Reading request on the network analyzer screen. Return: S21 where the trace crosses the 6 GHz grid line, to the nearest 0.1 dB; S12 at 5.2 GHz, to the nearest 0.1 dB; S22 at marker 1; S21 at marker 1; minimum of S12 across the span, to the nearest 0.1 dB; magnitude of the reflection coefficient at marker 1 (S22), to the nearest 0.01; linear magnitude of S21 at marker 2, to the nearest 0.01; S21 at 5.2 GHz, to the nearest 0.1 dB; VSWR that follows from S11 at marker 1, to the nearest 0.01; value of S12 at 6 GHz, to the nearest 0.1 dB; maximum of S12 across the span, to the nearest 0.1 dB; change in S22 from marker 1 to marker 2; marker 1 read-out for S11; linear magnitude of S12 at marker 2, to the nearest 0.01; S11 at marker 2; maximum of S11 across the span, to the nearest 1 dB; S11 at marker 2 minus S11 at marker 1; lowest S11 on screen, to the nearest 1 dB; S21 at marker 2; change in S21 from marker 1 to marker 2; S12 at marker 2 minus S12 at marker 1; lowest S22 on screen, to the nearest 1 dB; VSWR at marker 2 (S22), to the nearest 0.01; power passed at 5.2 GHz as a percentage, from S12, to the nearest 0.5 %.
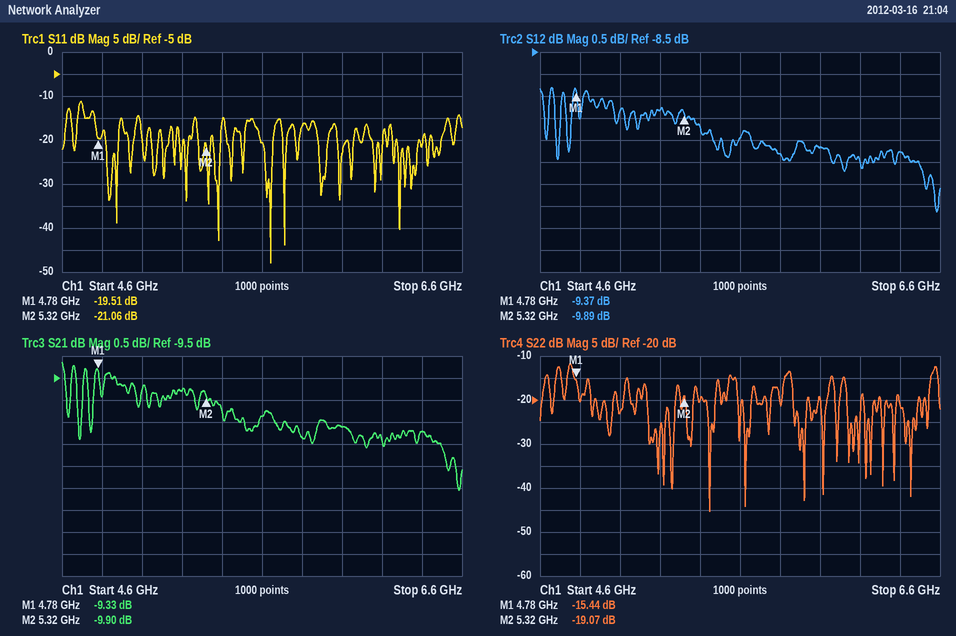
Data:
-10.6 dB
-9.8 dB
-15.44 dB
-9.33 dB
-12.1 dB
0.17
0.32
-9.8 dB
1.24
-10.7 dB
-9.3 dB
-3.63 dB
-19.51 dB
0.32
-21.06 dB
-11 dB
-1.55 dB
-48 dB
-9.90 dB
-0.57 dB
-0.52 dB
-45 dB
1.25
10.5 %
